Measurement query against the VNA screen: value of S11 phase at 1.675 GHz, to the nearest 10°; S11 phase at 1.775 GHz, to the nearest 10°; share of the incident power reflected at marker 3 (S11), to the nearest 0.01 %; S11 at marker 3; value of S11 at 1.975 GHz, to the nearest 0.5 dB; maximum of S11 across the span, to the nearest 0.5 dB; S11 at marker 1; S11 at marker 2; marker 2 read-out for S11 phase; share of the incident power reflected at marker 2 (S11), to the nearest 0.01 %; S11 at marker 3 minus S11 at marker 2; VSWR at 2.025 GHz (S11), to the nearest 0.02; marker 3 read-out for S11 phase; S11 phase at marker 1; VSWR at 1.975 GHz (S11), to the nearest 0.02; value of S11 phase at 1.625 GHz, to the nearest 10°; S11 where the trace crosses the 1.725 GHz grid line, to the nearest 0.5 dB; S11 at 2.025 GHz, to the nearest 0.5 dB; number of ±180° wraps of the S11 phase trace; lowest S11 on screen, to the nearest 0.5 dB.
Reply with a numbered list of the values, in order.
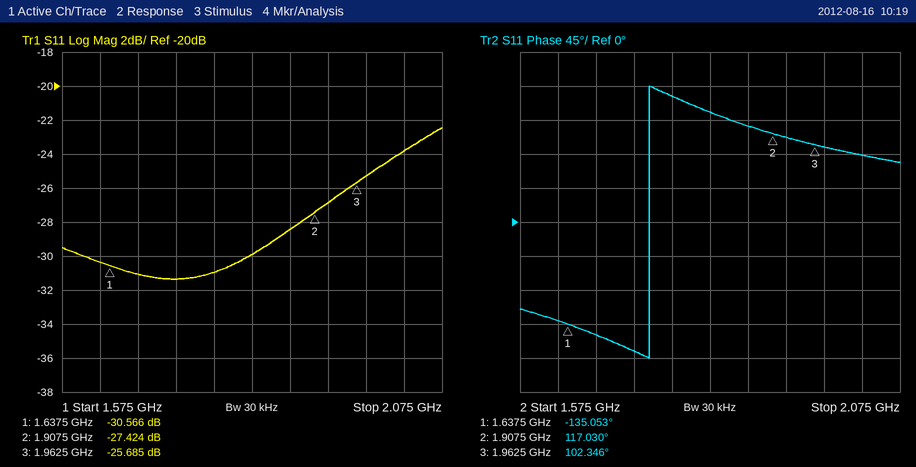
1. -150°
2. 170°
3. 0.27 %
4. -25.685 dB
5. -25.5 dB
6. -22.5 dB
7. -30.566 dB
8. -27.424 dB
9. 117.030°
10. 0.18 %
11. 1.739 dB
12. 1.14
13. 102.346°
14. -135.053°
15. 1.12
16. -130°
17. -31.5 dB
18. -24.0 dB
19. 1
20. -31.5 dB
